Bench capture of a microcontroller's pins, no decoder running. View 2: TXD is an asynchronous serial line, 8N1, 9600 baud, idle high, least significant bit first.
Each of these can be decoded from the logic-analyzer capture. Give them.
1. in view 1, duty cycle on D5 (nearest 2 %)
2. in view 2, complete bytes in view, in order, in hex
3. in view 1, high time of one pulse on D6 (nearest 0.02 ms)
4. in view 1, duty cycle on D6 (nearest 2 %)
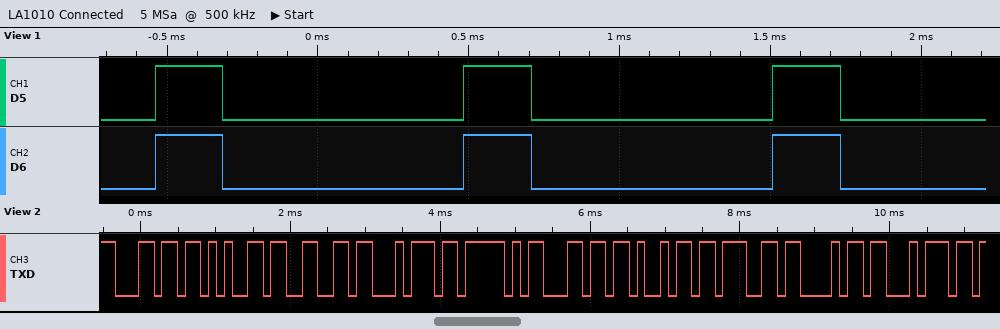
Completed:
22 %
0x6C 0x65 0x66 0x74 0x5F 0x6C 0x69 0x67 0x68 0x74
0.22 ms
22 %
